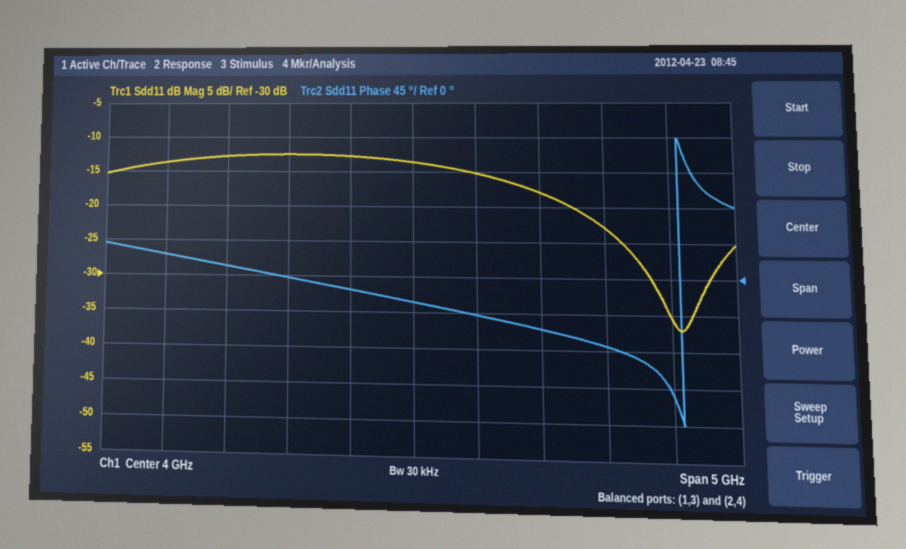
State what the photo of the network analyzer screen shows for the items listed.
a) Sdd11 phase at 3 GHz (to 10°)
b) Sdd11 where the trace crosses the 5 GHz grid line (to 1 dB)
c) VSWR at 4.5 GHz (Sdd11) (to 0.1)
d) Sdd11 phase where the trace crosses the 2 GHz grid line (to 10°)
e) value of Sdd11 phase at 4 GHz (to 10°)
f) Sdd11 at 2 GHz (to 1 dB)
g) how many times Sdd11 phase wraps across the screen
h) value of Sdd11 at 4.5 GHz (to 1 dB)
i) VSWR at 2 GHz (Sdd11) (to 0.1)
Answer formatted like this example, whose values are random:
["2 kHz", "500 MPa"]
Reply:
["0°", "-18 dB", "1.4", "30°", "-30°", "-14 dB", "1", "-15 dB", "1.5"]
